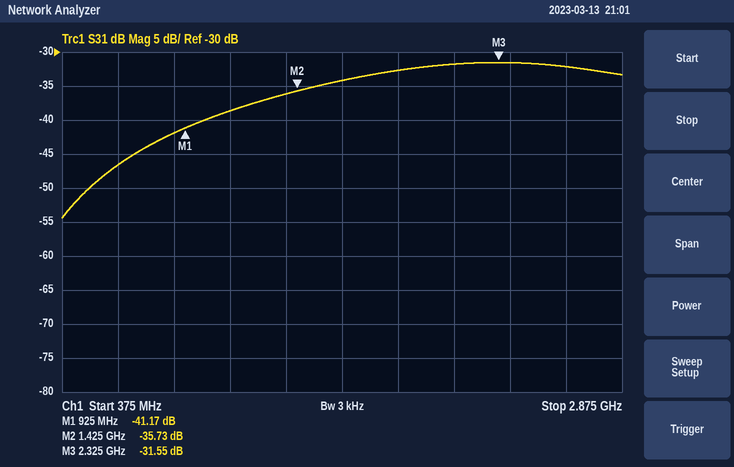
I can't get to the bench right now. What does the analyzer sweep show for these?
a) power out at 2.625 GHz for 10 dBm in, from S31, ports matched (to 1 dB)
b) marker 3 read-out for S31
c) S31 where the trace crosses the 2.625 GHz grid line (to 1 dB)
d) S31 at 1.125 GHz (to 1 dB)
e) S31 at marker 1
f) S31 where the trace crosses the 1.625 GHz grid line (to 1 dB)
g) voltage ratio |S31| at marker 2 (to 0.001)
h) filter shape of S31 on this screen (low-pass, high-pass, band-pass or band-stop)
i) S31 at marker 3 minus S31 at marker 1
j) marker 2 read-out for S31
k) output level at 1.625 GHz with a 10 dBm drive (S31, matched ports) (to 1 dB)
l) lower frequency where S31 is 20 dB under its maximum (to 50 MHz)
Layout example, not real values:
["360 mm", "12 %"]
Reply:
["-22 dBm", "-31.55 dB", "-32 dB", "-39 dB", "-41.17 dB", "-34 dB", "0.016", "high-pass", "9.62 dB", "-35.73 dB", "-24 dBm", "450 MHz"]
